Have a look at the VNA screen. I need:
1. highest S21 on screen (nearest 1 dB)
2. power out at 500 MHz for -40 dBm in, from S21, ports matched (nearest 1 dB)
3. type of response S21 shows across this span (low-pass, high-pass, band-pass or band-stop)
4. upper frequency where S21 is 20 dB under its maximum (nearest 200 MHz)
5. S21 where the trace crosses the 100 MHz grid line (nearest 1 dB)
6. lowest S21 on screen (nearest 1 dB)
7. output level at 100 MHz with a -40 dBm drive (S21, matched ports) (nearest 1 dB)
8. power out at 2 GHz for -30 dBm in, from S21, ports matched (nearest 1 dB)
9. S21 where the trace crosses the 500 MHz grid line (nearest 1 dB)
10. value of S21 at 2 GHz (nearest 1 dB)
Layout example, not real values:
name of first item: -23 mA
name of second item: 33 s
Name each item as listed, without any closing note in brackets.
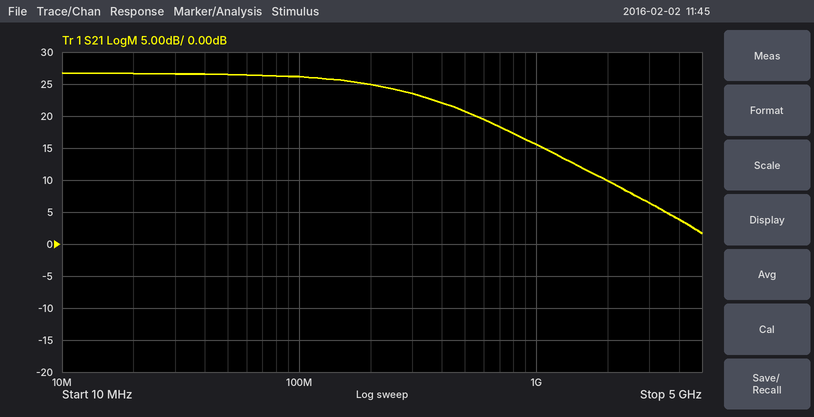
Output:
highest S21 on screen: 27 dB
power out at 500 MHz for -40 dBm in, from S21, ports matched: -19 dBm
type of response S21 shows across this span: low-pass
upper frequency where S21 is 20 dB under its maximum: 2.8 GHz
S21 where the trace crosses the 100 MHz grid line: 26 dB
lowest S21 on screen: 2 dB
output level at 100 MHz with a -40 dBm drive (S21, matched ports): -14 dBm
power out at 2 GHz for -30 dBm in, from S21, ports matched: -20 dBm
S21 where the trace crosses the 500 MHz grid line: 21 dB
value of S21 at 2 GHz: 10 dB
